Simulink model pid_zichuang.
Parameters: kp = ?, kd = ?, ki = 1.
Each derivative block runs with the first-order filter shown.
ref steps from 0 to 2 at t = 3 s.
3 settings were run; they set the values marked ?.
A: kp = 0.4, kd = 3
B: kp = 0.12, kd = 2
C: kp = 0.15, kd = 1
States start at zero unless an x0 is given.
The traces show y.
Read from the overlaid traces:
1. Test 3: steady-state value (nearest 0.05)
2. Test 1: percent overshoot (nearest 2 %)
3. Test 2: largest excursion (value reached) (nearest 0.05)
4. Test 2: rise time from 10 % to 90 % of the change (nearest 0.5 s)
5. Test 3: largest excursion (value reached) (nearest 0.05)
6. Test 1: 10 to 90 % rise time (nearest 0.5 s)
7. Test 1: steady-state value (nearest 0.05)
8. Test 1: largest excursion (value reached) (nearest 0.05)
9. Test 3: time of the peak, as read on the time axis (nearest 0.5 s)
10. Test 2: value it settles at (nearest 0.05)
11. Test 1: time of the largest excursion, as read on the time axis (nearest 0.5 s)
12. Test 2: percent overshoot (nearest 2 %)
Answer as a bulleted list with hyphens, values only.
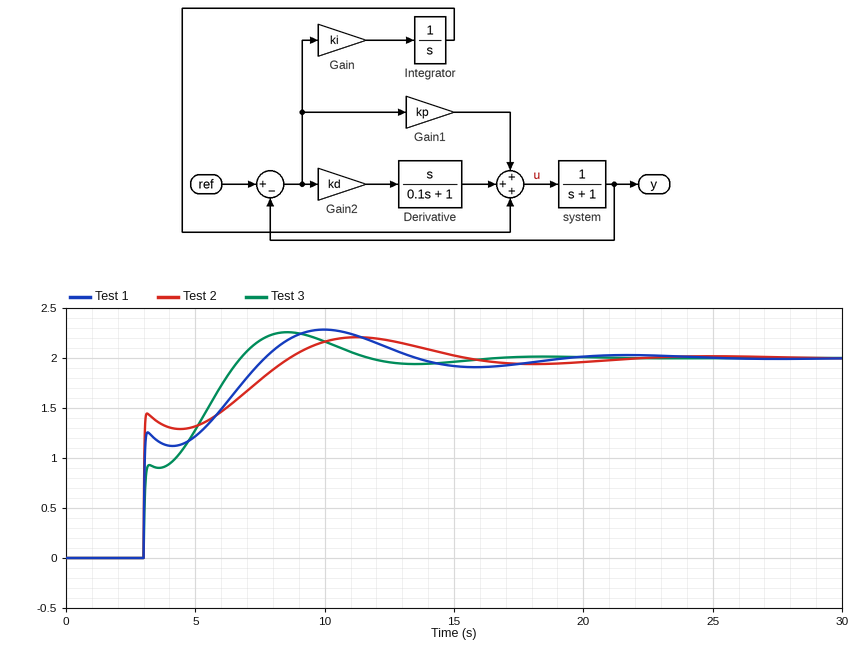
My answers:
- 2.00
- 14 %
- 2.20
- 4.5 s
- 2.25
- 4.0 s
- 2.00
- 2.30
- 8.5 s
- 2.00
- 10.0 s
- 10 %
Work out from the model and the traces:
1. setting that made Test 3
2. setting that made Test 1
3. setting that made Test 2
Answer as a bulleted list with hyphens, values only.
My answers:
- C
- B
- A
